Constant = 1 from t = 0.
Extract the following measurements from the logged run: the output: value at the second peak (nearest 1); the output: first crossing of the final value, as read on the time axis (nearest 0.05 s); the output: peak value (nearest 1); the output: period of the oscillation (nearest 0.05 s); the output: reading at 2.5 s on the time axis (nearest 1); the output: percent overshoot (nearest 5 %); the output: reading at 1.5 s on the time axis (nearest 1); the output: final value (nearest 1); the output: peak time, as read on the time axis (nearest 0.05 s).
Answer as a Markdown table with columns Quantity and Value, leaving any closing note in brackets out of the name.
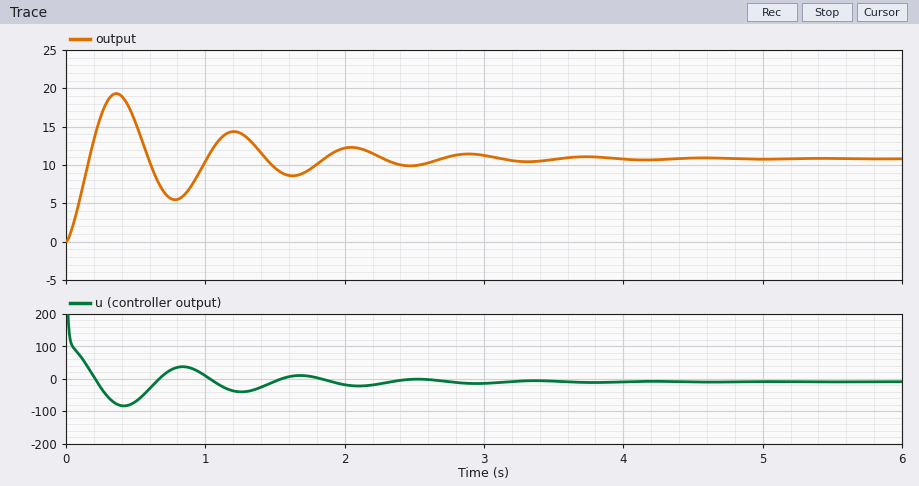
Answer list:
| Quantity | Value |
|---|---|
| the output: value at the second peak | 14 |
| the output: first crossing of the final value, as read on the time axis | 0.15 s |
| the output: peak value | 19 |
| the output: period of the oscillation | 0.85 s |
| the output: reading at 2.5 s on the time axis | 10 |
| the output: percent overshoot | 80 % |
| the output: reading at 1.5 s on the time axis | 10 |
| the output: final value | 11 |
| the output: peak time, as read on the time axis | 0.35 s |
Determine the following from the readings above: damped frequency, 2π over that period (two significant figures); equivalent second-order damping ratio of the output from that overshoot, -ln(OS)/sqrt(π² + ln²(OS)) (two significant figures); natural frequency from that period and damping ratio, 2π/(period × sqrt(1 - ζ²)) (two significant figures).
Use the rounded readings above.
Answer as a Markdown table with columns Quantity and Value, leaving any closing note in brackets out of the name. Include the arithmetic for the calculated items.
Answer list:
| Quantity | Value |
|---|---|
| damped frequency, 2π over that period | 2π / 0.85 = 7.4 rad/s |
| equivalent second-order damping ratio of the output from that overshoot, -ln(OS)/sqrt(π² + ln²(OS)) | ln(0.8) = -0.223; 0.223 / sqrt(9.870 + 0.050) = 0.071 |
| natural frequency from that period and damping ratio, 2π/(period × sqrt(1 - ζ²)) | 2π / (0.85 × sqrt(1 - 0.071²)) = 7.4 rad/s |
